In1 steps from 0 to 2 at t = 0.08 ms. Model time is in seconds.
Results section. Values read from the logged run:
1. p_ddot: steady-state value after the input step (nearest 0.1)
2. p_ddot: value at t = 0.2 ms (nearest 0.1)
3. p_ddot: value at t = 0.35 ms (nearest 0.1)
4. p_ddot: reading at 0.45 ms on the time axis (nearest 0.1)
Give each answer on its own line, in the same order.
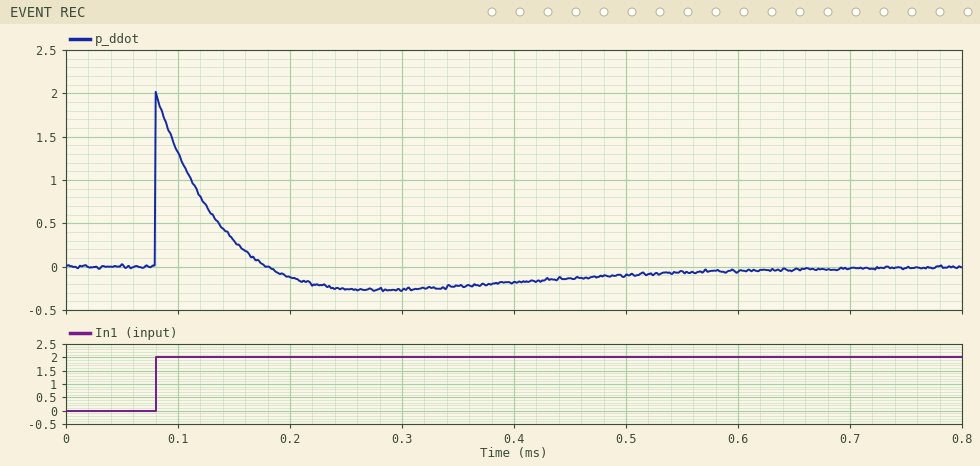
0.0
-0.1
-0.2
-0.1
